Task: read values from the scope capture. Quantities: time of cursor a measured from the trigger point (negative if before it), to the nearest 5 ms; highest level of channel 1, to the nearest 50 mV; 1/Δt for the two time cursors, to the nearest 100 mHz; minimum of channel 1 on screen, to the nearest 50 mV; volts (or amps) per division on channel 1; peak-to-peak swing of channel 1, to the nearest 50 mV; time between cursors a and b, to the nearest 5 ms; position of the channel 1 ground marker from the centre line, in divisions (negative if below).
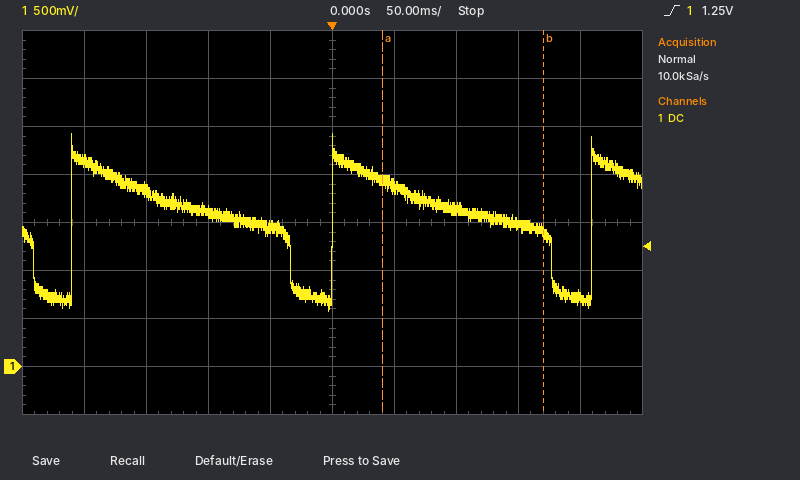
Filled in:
+40 ms
2.45 V
7.7 Hz
600 mV
500 mV
1.85 V
130 ms
-3.0 div
